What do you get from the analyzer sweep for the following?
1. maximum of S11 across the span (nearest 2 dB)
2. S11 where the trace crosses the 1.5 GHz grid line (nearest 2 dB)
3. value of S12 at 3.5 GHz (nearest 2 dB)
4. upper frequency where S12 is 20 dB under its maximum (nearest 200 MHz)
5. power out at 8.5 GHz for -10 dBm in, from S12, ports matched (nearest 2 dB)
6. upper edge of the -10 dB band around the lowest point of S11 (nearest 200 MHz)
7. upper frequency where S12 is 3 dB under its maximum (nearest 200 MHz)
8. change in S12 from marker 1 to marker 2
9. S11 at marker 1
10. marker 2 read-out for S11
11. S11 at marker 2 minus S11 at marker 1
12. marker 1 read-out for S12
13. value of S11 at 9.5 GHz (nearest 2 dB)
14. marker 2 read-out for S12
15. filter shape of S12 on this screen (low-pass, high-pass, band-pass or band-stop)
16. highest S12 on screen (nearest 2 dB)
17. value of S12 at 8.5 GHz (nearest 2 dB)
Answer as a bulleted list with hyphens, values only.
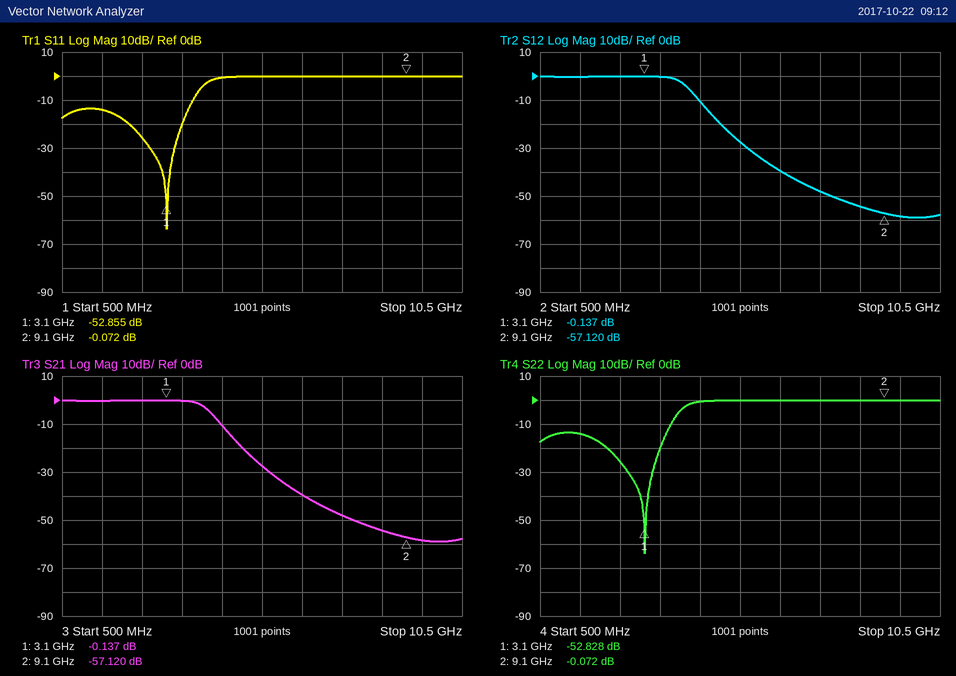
- 0 dB
- -14 dB
- 0 dB
- 5.0 GHz
- -64 dBm
- 3.8 GHz
- 4.0 GHz
- -56.983 dB
- -52.855 dB
- -0.072 dB
- 52.783 dB
- -0.137 dB
- 0 dB
- -57.120 dB
- low-pass
- 0 dB
- -54 dB
